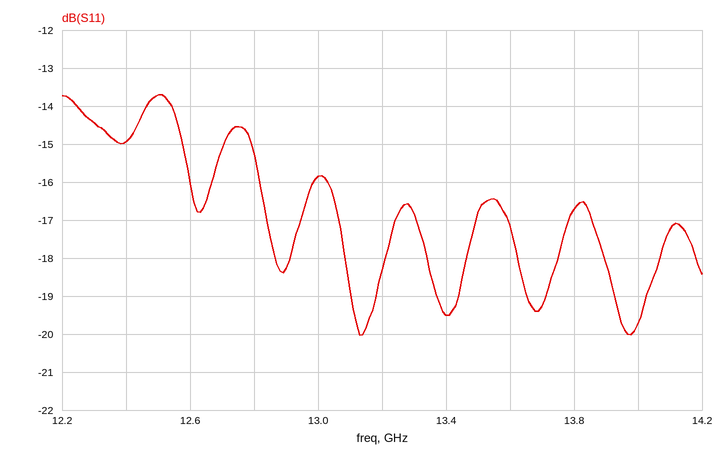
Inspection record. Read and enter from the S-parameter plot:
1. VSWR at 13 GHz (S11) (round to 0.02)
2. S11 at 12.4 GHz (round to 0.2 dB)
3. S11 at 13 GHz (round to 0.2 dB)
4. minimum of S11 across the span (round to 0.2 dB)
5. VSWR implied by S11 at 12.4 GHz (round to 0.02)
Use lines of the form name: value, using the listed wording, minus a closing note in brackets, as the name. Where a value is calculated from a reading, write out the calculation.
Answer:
VSWR at 13 GHz (S11): |Γ| = 10^(-15.8/20) = 0.1622; VSWR = (1 + 0.1622)/(1 − 0.1622) ≈ 1.39, so 1.38 to the nearest 0.02
S11 at 12.4 GHz: -15.0 dB
S11 at 13 GHz: -15.8 dB
minimum of S11 across the span: -20.0 dB
VSWR implied by S11 at 12.4 GHz: |Γ| = 10^(-15/20) = 0.1778; VSWR = (1 + 0.1778)/(1 − 0.1778) ≈ 1.43, so 1.44 to the nearest 0.02
